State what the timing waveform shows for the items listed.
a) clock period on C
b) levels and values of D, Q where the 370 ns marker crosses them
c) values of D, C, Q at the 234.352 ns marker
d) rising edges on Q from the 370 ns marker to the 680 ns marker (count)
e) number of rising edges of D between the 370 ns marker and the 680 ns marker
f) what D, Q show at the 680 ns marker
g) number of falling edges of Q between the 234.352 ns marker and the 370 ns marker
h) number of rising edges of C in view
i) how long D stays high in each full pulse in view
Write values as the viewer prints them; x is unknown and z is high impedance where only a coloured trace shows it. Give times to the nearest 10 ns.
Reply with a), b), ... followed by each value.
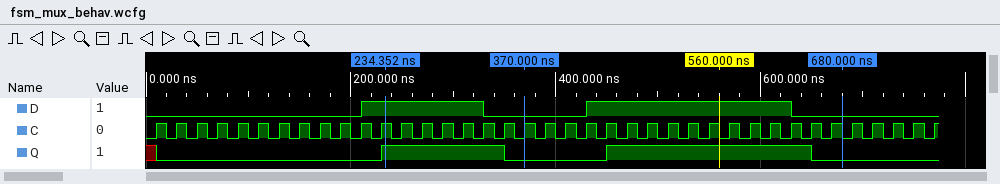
a) 20 ns
b) D=0, Q=0
c) D=1, C=1, Q=1
d) 1
e) 1
f) D=0, Q=0
g) 1
h) 39
i) 120 ns, 200 ns
